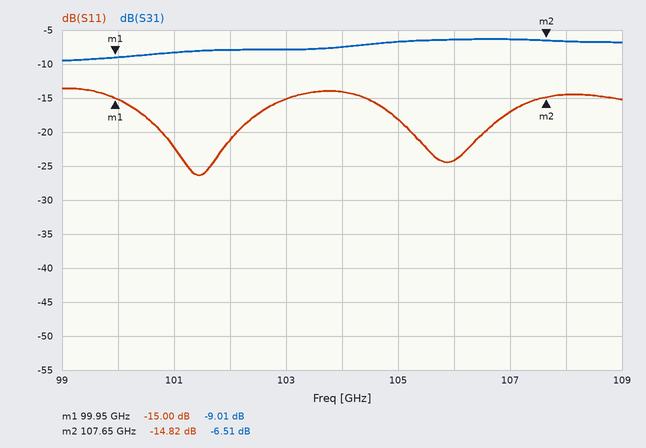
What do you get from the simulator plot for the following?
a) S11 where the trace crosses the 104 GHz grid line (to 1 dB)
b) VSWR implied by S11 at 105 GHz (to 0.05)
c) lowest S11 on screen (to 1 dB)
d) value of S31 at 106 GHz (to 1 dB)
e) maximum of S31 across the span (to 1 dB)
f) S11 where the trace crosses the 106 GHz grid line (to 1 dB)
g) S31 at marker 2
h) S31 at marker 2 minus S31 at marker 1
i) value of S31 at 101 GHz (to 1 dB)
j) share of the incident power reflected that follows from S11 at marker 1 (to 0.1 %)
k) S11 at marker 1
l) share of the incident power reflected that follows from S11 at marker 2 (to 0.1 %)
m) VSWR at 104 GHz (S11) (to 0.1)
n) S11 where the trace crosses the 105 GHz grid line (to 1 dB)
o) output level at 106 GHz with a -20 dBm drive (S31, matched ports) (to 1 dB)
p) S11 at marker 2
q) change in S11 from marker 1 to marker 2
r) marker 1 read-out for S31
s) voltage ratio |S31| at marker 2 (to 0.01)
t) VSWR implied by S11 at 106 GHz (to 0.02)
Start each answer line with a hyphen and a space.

- -14 dB
- 1.30
- -26 dB
- -6 dB
- -6 dB
- -24 dB
- -6.51 dB
- 2.50 dB
- -8 dB
- 3.2 %
- -15.00 dB
- 3.3 %
- 1.5
- -18 dB
- -26 dBm
- -14.82 dB
- 0.18 dB
- -9.01 dB
- 0.47
- 1.14
